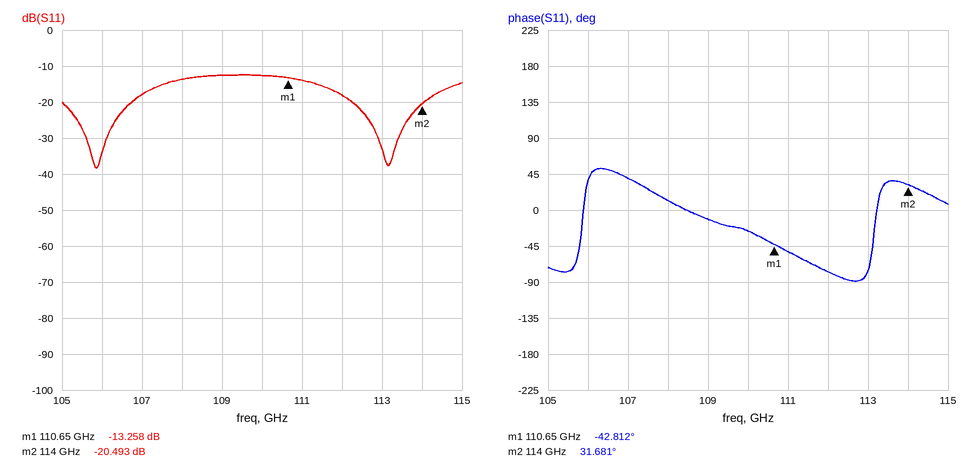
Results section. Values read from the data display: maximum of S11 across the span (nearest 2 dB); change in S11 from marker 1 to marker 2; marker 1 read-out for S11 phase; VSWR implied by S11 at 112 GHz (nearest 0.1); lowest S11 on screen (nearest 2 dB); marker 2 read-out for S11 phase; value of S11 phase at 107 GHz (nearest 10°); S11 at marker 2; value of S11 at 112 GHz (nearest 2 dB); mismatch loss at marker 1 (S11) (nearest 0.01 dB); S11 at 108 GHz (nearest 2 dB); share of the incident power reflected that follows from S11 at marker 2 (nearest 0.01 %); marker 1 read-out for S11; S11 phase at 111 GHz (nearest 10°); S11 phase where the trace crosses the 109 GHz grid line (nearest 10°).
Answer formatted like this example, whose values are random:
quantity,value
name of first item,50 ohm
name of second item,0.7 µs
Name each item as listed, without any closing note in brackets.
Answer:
quantity,value
maximum of S11 across the span,-12 dB
change in S11 from marker 1 to marker 2,-7.235 dB
marker 1 read-out for S11 phase,-42.812°
VSWR implied by S11 at 112 GHz,1.3
lowest S11 on screen,-38 dB
marker 2 read-out for S11 phase,31.681°
value of S11 phase at 107 GHz,40°
S11 at marker 2,-20.493 dB
value of S11 at 112 GHz,-18 dB
mismatch loss at marker 1 (S11),0.21 dB
S11 at 108 GHz,-14 dB
share of the incident power reflected that follows from S11 at marker 2,0.89 %
marker 1 read-out for S11,-13.258 dB
S11 phase at 111 GHz,-50°
S11 phase where the trace crosses the 109 GHz grid line,-10°
